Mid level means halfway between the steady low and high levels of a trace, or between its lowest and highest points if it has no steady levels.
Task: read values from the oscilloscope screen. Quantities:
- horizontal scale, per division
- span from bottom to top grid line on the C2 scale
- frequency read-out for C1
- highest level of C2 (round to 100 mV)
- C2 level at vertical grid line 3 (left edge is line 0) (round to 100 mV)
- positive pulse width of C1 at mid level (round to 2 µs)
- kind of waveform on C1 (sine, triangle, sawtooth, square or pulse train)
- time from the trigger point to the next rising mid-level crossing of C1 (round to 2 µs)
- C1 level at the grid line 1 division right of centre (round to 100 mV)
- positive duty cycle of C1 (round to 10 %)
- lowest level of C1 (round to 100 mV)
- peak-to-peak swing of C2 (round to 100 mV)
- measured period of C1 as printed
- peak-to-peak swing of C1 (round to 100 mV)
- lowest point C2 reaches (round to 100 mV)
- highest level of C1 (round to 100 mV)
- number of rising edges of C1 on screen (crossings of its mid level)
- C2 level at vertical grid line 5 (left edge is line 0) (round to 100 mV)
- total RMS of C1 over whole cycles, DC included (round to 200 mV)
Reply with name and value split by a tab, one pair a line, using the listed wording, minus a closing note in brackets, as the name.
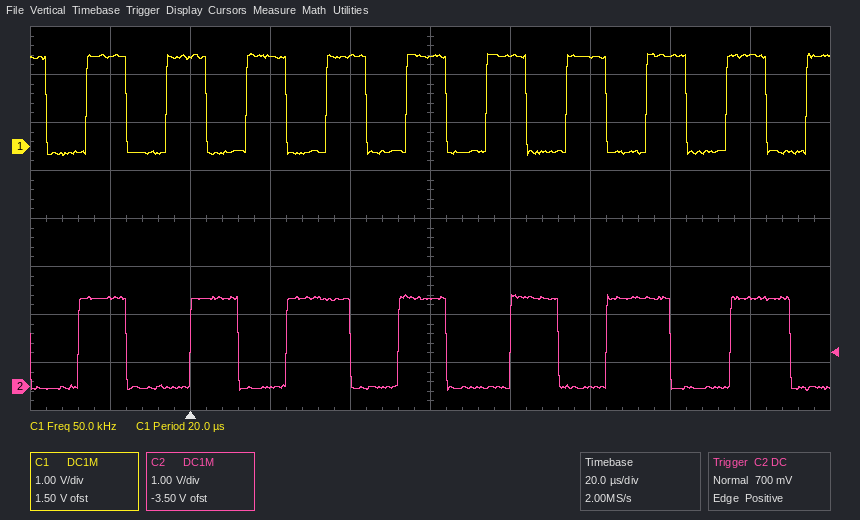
horizontal scale, per division	20 µs
span from bottom to top grid line on the C2 scale	8 V
frequency read-out for C1	50.0 kHz
highest level of C2	1.9 V
C2 level at vertical grid line 3 (left edge is line 0)	0.0 V
positive pulse width of C1 at mid level	10 µs
kind of waveform on C1	square
time from the trigger point to the next rising mid-level crossing of C1	14 µs
C1 level at the grid line 1 division right of centre	1.9 V
positive duty cycle of C1	50 %
lowest level of C1	-200 mV
peak-to-peak swing of C2	2.0 V
measured period of C1 as printed	20.0 µs
peak-to-peak swing of C1	2.1 V
lowest point C2 reaches	-100 mV
highest level of C1	1.9 V
number of rising edges of C1 on screen	10
C2 level at vertical grid line 5 (left edge is line 0)	1.8 V
total RMS of C1 over whole cycles, DC included	1.4 V
